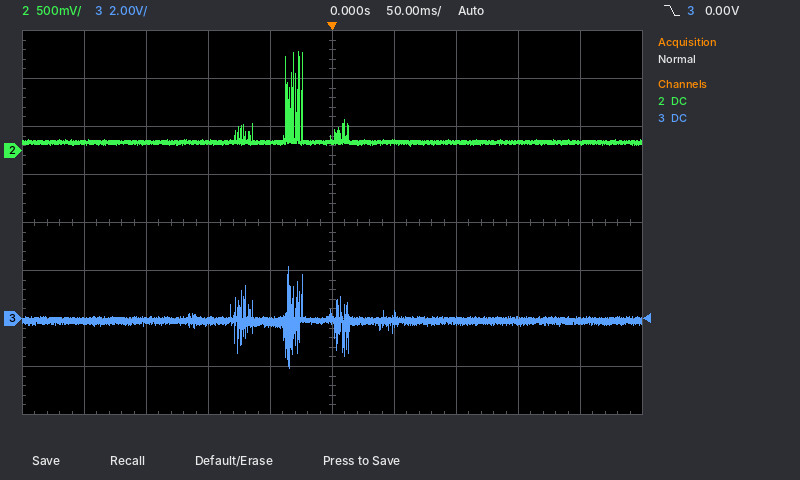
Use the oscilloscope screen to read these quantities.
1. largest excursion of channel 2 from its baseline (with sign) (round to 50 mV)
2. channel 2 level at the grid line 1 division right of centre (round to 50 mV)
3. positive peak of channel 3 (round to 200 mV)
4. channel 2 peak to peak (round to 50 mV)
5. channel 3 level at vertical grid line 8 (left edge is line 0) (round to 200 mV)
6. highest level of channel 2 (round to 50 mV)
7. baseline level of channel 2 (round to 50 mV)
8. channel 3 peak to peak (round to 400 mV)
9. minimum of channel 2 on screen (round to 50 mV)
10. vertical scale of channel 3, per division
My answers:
+950 mV
100 mV
2.2 V
1.00 V
-200 mV
1.05 V
100 mV
4.4 V
50 mV
2 V
